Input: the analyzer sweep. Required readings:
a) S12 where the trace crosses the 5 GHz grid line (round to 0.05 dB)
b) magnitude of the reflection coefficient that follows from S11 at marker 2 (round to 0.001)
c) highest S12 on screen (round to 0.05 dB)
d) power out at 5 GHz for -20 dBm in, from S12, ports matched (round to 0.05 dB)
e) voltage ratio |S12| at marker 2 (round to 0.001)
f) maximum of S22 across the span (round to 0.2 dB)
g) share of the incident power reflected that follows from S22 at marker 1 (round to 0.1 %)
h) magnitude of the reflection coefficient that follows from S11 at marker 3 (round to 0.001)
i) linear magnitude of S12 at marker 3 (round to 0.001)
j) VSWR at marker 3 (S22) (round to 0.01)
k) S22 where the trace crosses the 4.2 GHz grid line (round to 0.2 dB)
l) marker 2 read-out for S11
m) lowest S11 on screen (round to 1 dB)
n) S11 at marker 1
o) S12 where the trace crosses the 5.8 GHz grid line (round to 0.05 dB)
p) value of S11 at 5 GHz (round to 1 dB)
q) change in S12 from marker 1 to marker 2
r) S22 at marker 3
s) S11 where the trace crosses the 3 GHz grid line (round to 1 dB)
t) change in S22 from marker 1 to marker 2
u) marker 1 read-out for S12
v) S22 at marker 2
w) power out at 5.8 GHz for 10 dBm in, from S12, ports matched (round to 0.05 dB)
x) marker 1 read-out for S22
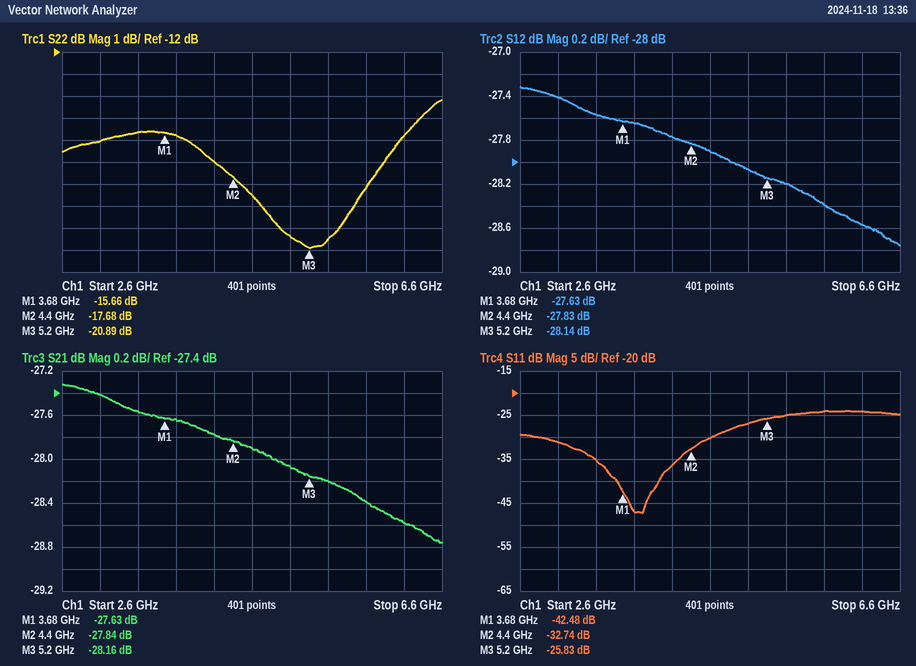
-28.05 dB
0.023
-27.30 dB
-48.05 dBm
0.041
-14.2 dB
2.7 %
0.051
0.039
1.20
-17.0 dB
-32.74 dB
-47 dB
-42.48 dB
-28.40 dB
-27 dB
-0.20 dB
-20.89 dB
-31 dB
-2.02 dB
-27.63 dB
-17.68 dB
-18.40 dBm
-15.66 dB
